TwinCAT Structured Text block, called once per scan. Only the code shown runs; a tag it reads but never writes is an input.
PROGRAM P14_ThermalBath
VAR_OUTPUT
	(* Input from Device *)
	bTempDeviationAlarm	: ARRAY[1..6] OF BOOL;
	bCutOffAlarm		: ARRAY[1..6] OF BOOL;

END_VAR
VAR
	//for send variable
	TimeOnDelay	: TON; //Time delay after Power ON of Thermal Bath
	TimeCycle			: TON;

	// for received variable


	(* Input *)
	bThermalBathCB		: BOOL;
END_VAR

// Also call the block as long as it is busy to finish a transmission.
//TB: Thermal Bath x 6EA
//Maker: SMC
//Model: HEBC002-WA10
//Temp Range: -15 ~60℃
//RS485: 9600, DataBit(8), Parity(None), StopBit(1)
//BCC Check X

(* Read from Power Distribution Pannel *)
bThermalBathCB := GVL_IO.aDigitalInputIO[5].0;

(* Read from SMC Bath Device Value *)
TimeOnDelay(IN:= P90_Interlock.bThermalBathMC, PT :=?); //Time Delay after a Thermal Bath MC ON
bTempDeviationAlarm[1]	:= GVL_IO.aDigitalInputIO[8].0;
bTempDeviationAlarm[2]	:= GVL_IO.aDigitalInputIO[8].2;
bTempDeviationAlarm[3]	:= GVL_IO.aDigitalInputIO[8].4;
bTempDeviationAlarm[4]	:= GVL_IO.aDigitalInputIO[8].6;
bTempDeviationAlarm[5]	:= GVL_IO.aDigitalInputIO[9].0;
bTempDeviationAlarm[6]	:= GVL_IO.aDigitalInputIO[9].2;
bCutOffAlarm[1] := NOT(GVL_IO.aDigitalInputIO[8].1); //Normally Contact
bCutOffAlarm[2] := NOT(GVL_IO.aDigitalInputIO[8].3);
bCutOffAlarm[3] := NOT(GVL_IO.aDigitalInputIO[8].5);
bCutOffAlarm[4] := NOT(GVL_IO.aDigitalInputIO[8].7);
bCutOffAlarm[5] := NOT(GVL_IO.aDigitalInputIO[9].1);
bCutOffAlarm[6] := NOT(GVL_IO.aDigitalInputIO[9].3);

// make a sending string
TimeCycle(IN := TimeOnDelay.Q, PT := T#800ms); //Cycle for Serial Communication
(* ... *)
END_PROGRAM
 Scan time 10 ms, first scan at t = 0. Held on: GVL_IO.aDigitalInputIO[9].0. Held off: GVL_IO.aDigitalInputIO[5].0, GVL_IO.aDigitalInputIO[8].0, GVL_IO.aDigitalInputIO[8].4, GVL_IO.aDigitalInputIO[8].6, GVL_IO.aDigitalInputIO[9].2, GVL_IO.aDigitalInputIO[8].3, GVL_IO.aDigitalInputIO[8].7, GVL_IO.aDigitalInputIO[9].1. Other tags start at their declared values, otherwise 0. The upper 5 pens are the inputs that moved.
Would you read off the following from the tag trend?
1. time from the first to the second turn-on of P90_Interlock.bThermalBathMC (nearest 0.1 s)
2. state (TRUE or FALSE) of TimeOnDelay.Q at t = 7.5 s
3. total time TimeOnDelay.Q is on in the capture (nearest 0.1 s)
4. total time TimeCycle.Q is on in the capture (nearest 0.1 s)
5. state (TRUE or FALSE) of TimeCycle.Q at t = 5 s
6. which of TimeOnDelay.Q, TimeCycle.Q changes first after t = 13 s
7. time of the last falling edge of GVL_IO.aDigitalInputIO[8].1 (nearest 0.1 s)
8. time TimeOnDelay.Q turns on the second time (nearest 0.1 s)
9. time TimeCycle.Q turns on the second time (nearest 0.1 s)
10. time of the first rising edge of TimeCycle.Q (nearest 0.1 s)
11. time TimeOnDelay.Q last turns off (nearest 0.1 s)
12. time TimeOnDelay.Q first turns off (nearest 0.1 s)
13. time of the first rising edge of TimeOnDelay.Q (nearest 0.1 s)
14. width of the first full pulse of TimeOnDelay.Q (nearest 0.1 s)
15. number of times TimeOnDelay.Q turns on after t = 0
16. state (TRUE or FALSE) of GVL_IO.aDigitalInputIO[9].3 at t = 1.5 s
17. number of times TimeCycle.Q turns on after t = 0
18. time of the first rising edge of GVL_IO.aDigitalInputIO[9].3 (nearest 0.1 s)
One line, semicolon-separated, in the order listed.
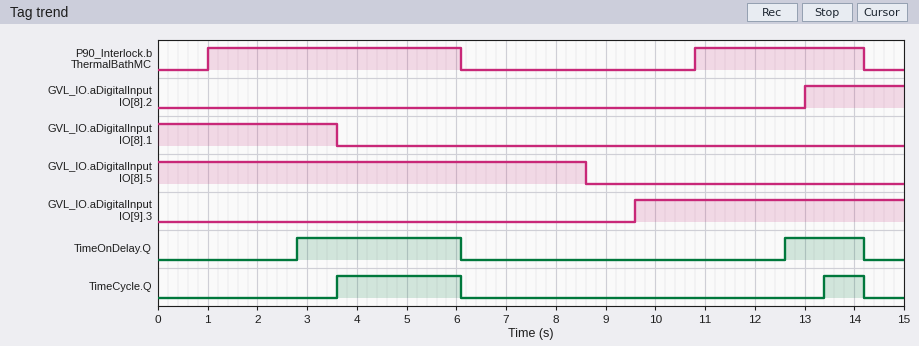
9.8 s; FALSE; 4.9 s; 3.3 s; TRUE; TimeCycle.Q; 3.6 s; 12.6 s; 13.4 s; 3.6 s; 14.2 s; 6.1 s; 2.8 s; 3.3 s; 2; FALSE; 2; 9.6 s
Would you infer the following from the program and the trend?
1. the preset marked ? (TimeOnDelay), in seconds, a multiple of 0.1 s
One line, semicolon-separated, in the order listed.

1.8 s
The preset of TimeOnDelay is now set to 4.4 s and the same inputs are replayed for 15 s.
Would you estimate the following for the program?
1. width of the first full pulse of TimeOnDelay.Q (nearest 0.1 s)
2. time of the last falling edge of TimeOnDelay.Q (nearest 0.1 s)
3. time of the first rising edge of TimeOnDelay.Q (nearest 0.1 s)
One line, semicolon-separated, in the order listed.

0.7 s; 6.1 s; 5.4 s
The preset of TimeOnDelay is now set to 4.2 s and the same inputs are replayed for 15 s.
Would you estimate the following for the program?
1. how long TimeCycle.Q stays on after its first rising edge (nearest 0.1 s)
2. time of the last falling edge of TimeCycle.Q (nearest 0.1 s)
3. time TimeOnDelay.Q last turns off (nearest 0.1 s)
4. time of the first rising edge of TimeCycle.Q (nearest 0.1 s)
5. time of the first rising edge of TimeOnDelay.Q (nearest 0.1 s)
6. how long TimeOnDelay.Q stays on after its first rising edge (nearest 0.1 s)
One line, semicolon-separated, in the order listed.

0.1 s; 6.1 s; 6.1 s; 6.0 s; 5.2 s; 0.9 s
